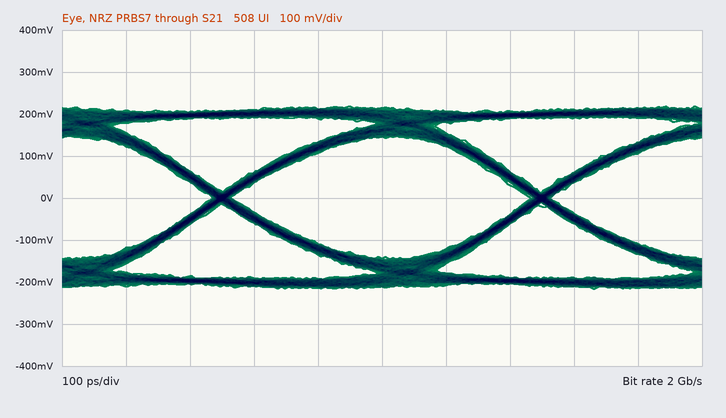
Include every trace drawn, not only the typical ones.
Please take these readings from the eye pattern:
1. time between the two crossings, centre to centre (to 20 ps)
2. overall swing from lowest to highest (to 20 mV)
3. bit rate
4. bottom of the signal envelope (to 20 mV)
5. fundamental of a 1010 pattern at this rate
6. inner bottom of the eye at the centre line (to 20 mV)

500 ps
440 mV
2 Gb/s
-220 mV
1 GHz
-140 mV
